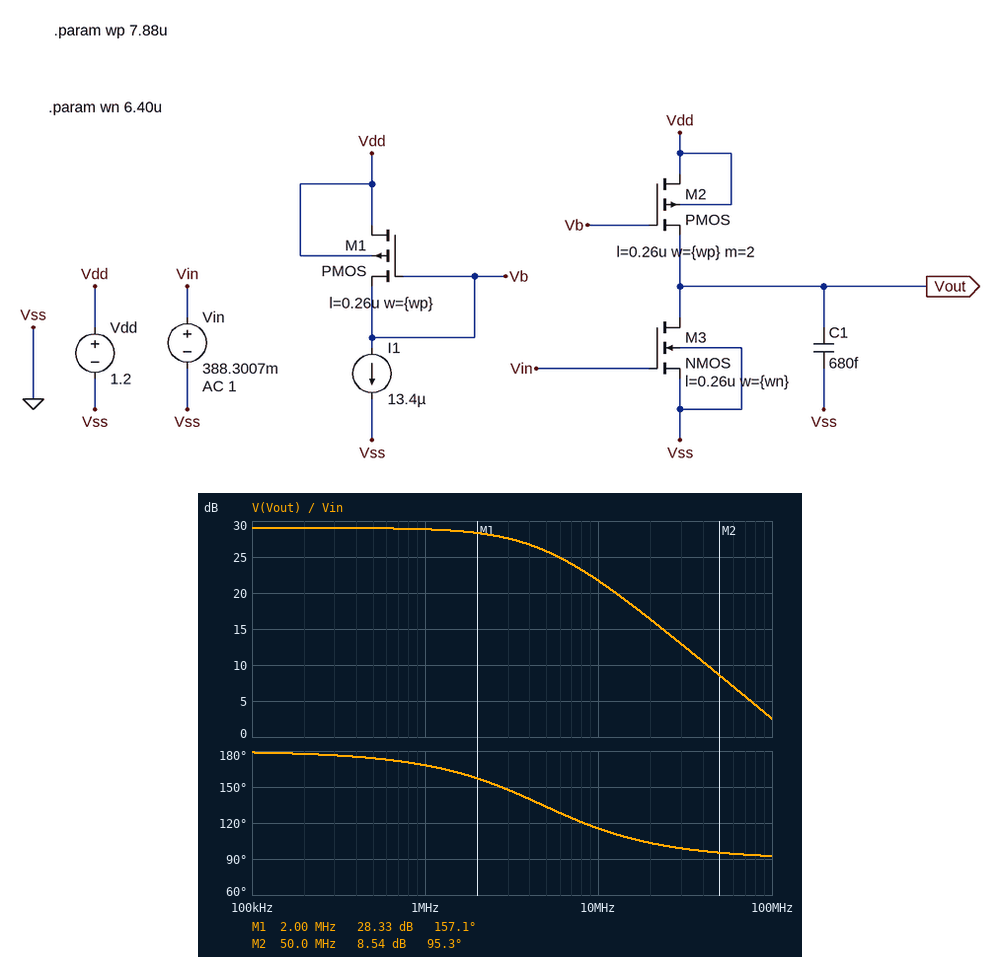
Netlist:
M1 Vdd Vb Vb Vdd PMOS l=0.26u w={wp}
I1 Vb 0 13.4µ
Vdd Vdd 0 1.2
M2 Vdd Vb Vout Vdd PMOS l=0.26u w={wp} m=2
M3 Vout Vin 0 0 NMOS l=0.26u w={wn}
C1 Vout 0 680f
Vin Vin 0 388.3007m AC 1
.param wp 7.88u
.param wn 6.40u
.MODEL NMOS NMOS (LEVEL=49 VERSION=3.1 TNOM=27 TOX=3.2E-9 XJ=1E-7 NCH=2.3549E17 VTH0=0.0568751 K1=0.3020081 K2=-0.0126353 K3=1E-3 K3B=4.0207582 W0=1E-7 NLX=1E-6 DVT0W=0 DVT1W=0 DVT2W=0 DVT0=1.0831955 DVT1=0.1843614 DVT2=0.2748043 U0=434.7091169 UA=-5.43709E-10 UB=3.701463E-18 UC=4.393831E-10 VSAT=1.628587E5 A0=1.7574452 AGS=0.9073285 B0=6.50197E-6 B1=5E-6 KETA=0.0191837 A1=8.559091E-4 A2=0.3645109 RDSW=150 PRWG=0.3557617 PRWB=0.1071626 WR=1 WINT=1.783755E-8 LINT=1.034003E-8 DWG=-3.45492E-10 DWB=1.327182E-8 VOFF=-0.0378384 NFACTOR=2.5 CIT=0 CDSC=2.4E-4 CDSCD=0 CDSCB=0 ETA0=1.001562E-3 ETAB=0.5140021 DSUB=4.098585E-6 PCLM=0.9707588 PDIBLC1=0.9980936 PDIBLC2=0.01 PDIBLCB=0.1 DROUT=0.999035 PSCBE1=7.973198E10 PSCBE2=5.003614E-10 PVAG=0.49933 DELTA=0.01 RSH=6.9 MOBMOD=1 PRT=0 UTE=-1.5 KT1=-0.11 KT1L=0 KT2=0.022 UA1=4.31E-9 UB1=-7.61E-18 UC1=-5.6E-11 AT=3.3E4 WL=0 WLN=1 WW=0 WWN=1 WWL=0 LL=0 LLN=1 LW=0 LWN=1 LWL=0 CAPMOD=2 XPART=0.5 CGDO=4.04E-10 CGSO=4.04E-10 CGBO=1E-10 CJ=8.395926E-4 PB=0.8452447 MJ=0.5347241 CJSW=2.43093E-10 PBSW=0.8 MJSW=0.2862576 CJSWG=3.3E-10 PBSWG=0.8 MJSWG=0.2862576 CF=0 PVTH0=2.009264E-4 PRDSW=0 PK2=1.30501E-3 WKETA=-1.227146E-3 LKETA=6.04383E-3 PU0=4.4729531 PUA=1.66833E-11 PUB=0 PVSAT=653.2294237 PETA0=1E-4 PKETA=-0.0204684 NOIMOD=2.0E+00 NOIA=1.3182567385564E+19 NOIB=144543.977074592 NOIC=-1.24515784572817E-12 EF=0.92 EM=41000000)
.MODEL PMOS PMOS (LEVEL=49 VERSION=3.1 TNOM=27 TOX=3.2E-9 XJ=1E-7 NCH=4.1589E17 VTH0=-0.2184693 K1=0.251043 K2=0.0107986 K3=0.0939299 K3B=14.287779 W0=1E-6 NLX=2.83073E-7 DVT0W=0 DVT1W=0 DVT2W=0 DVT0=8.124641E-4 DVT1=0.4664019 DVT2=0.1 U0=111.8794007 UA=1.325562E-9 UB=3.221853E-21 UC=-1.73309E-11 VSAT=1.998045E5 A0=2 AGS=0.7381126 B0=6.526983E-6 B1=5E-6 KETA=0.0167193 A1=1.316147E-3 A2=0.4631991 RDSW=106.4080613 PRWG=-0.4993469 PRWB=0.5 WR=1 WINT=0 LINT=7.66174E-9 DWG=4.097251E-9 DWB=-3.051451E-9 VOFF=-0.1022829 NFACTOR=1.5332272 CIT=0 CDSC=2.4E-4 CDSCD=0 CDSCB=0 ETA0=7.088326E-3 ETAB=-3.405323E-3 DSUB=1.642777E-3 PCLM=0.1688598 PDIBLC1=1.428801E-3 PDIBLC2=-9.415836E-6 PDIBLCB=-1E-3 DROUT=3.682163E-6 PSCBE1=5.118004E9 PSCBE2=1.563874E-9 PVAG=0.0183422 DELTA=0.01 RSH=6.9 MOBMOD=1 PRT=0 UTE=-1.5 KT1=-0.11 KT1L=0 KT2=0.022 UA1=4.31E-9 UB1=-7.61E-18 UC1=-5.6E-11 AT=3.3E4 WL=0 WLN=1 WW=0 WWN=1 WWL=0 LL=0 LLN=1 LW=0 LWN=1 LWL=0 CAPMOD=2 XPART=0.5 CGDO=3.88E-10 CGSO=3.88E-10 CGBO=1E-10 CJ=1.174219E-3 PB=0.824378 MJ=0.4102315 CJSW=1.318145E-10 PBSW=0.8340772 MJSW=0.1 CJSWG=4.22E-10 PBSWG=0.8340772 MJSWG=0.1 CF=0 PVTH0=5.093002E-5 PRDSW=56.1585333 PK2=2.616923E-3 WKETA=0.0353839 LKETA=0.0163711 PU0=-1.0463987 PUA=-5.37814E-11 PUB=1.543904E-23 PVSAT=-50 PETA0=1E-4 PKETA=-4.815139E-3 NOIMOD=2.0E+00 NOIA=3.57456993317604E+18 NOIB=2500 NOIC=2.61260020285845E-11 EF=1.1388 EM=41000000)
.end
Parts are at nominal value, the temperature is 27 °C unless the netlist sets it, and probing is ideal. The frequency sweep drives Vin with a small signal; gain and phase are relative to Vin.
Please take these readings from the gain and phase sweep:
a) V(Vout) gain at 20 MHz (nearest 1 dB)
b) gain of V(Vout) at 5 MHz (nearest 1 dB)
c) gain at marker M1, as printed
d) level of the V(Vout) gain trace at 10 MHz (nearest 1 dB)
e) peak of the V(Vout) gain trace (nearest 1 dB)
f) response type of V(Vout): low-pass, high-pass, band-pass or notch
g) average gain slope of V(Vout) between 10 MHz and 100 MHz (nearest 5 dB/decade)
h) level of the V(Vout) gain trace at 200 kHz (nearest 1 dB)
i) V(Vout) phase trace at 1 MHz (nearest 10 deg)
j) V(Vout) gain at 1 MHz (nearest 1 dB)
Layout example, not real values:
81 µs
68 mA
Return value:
16 dB
26 dB
28.33 dB
22 dB
29 dB
low-pass
-20 dB/decade
29 dB
170 deg
29 dB
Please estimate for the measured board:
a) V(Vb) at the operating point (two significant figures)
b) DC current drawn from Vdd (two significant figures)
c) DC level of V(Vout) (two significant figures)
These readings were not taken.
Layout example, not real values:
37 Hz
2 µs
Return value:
800 mV
42 µA
610 mV
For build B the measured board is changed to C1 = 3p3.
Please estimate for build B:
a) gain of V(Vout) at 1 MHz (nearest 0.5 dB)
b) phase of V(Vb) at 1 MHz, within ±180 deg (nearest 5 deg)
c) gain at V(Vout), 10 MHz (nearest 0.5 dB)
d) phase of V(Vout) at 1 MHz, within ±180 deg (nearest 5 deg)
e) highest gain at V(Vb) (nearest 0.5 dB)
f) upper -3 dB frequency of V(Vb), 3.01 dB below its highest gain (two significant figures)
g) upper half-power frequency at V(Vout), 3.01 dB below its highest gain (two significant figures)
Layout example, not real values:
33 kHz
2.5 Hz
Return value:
26.0 dB
-135 deg
9.0 dB
135 deg
-47.0 dB
620 MHz
1.0 MHz
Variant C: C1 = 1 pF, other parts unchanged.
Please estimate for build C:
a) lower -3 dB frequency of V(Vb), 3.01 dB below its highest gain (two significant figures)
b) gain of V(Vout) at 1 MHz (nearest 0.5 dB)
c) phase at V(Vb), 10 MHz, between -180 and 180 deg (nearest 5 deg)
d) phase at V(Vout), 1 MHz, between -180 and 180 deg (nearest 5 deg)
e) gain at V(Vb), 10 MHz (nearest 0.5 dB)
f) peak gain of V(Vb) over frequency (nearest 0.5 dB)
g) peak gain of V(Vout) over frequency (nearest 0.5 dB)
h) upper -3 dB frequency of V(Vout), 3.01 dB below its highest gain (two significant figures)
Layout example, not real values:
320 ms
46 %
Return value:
3.2 MHz
28.5 dB
-165 deg
165 deg
-37.5 dB
-37.0 dB
29.0 dB
3.3 MHz
